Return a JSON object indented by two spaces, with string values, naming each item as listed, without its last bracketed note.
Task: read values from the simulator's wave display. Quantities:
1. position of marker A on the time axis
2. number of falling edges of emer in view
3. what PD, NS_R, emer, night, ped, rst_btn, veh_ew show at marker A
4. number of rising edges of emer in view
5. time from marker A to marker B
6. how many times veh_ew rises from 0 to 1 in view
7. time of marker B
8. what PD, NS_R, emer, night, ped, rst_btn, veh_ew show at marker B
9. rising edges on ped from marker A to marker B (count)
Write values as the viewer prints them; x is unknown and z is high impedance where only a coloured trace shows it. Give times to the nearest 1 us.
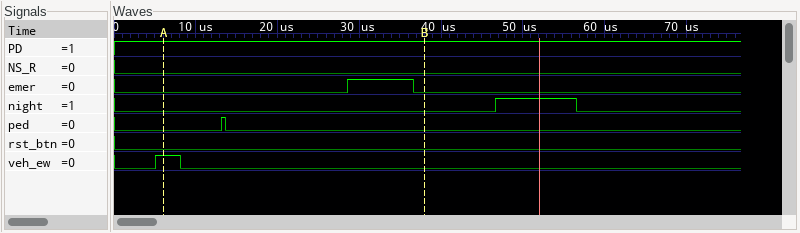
{
  "position of marker A on the time axis": "6 us",
  "number of falling edges of emer in view": "1",
  "what PD, NS_R, emer, night, ped, rst_btn, veh_ew show at marker A": "PD=1, NS_R=0, emer=0, night=0, ped=0, rst_btn=0, veh_ew=1",
  "number of rising edges of emer in view": "1",
  "time from marker A to marker B": "32 us",
  "how many times veh_ew rises from 0 to 1 in view": "1",
  "time of marker B": "38 us",
  "what PD, NS_R, emer, night, ped, rst_btn, veh_ew show at marker B": "PD=1, NS_R=0, emer=0, night=0, ped=0, rst_btn=0, veh_ew=0",
  "rising edges on ped from marker A to marker B": "1"
}
